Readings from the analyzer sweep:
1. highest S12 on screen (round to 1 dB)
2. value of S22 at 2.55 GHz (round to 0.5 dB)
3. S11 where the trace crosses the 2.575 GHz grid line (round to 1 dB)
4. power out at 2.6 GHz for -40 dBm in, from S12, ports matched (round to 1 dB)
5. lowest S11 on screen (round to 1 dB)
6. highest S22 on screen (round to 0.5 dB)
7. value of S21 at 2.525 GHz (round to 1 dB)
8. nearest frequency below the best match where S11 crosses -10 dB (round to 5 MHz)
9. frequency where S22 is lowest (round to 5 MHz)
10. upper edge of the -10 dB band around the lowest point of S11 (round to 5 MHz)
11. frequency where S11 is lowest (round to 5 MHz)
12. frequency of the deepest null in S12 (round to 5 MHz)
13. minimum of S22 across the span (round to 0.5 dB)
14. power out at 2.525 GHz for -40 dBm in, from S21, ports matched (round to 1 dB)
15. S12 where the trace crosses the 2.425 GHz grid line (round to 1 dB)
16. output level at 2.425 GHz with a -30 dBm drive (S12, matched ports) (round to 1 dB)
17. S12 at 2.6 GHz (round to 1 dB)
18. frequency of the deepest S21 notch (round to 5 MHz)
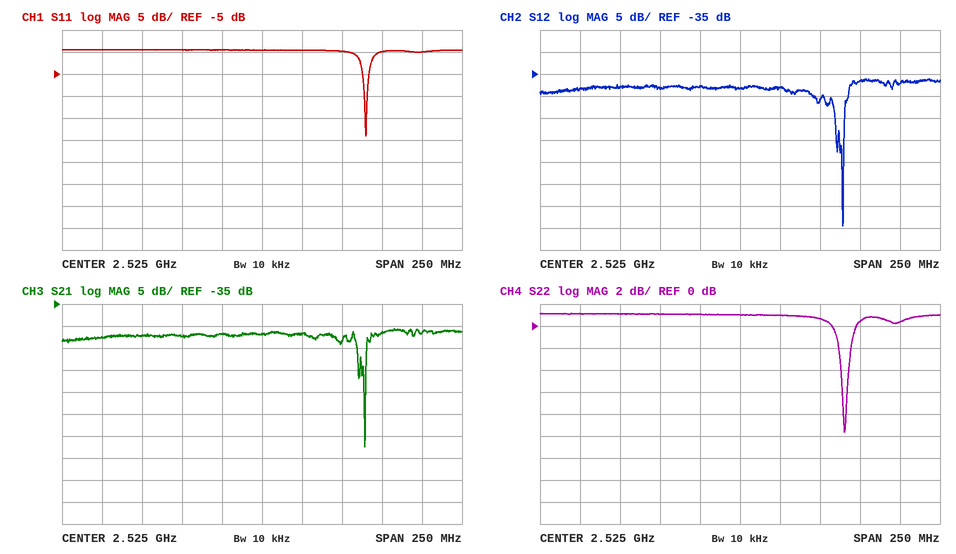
-36 dB
1.0 dB
0 dB
-77 dBm
-19 dB
1.0 dB
-42 dB
2.590 GHz
2.590 GHz
2.590 GHz
2.590 GHz
2.590 GHz
-9.5 dB
-82 dBm
-38 dB
-68 dBm
-37 dB
2.590 GHz
